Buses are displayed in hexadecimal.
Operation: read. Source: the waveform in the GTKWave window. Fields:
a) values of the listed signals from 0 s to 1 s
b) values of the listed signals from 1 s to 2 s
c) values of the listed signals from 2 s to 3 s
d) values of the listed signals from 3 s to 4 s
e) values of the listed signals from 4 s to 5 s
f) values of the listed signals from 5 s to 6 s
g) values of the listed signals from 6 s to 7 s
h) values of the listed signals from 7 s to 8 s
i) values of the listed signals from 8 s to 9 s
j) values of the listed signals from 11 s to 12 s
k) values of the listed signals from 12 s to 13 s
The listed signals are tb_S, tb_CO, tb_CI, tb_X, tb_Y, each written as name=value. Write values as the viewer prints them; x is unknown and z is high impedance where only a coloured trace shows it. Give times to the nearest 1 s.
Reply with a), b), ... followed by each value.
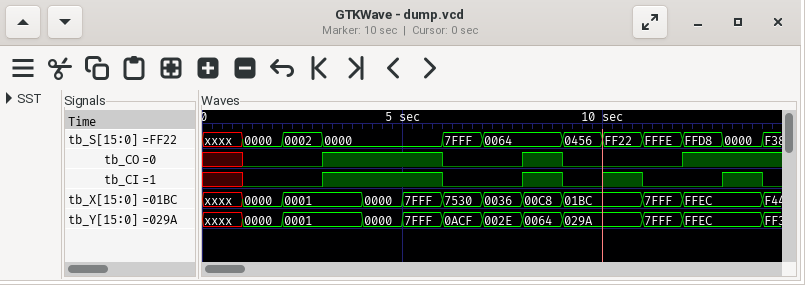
a) tb_S=xxxx, tb_CO=x, tb_CI=x, tb_X=xxxx, tb_Y=xxxx
b) tb_S=0000, tb_CO=0, tb_CI=0, tb_X=0000, tb_Y=0000
c) tb_S=0002, tb_CO=0, tb_CI=0, tb_X=0001, tb_Y=0001
d) tb_S=0000, tb_CO=1, tb_CI=1, tb_X=0001, tb_Y=0001
e) tb_S=0000, tb_CO=1, tb_CI=1, tb_X=0000, tb_Y=0000
f) tb_S=0000, tb_CO=1, tb_CI=1, tb_X=7FFF, tb_Y=7FFF
g) tb_S=7FFF, tb_CO=0, tb_CI=0, tb_X=7530, tb_Y=0ACF
h) tb_S=0064, tb_CO=0, tb_CI=0, tb_X=0036, tb_Y=002E
i) tb_S=0064, tb_CO=1, tb_CI=1, tb_X=00C8, tb_Y=0064
j) tb_S=FFFE, tb_CO=0, tb_CI=0, tb_X=7FFF, tb_Y=7FFF
k) tb_S=FFD8, tb_CO=1, tb_CI=0, tb_X=FFEC, tb_Y=FFEC
